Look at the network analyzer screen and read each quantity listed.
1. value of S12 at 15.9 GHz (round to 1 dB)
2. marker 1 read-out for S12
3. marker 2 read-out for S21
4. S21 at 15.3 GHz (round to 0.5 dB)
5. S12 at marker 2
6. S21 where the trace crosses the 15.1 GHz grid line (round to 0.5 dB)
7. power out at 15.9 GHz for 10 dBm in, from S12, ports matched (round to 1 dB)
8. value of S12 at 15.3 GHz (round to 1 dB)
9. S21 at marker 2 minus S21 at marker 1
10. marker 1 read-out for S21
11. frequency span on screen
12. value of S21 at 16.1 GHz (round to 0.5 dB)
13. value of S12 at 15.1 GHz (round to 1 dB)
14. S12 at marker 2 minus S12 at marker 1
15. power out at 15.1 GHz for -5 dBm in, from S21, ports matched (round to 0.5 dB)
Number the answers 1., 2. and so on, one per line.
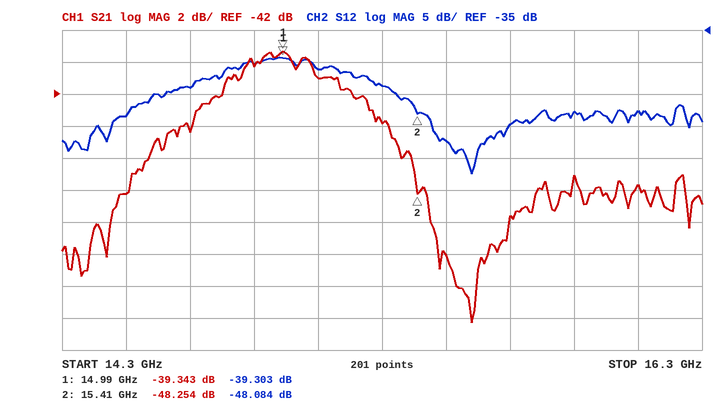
1. -48 dB
2. -39.303 dB
3. -48.254 dB
4. -44.0 dB
5. -48.084 dB
6. -41.0 dB
7. -38 dBm
8. -44 dB
9. -8.911 dB
10. -39.343 dB
11. 2 GHz
12. -47.5 dB
13. -41 dB
14. -8.781 dB
15. -46.0 dBm
